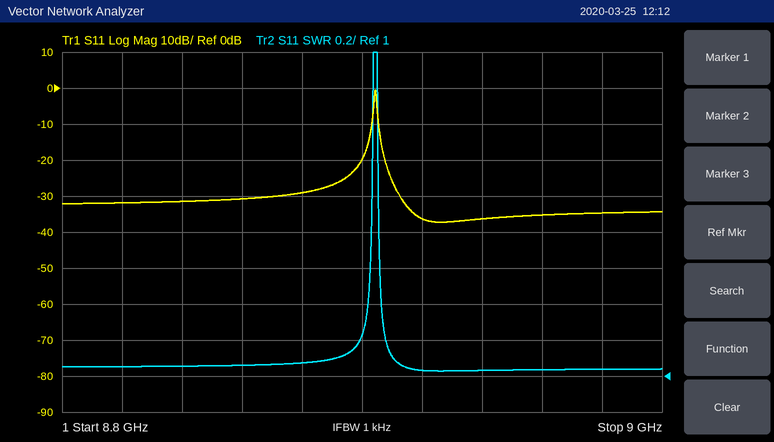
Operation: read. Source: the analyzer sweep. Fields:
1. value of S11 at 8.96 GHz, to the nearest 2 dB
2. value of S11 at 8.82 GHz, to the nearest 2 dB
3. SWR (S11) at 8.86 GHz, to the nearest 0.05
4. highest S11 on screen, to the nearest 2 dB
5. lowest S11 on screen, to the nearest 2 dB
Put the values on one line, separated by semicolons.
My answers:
-36 dB; -32 dB; 1.05; 0 dB; -38 dB
